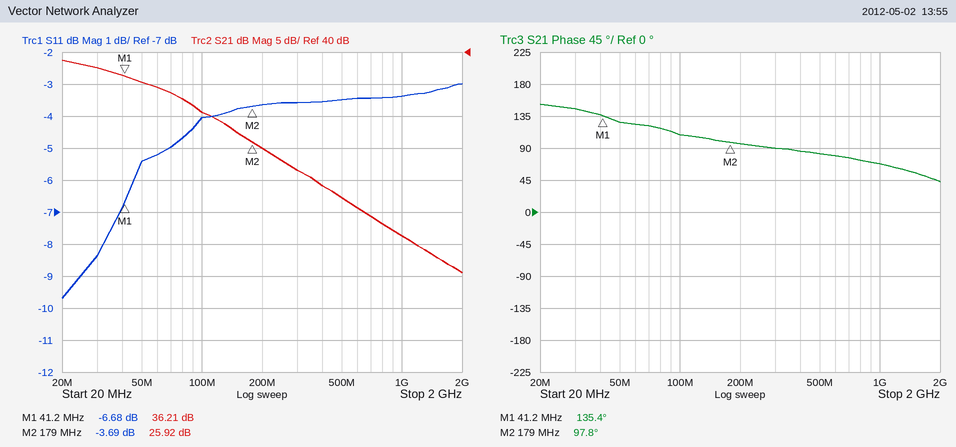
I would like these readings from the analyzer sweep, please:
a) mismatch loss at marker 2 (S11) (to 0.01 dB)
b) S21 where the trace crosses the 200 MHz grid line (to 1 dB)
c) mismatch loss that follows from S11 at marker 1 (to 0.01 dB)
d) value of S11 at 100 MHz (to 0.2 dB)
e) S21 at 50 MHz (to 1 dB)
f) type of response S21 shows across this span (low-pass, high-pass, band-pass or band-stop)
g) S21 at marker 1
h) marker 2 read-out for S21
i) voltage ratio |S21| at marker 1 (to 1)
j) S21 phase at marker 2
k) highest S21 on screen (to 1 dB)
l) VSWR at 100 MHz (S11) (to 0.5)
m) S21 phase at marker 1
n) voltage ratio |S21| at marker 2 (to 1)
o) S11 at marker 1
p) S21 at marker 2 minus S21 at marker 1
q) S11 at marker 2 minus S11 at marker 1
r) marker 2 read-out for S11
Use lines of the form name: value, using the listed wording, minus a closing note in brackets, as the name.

mismatch loss at marker 2 (S11): 2.42 dB
S21 where the trace crosses the 200 MHz grid line: 25 dB
mismatch loss that follows from S11 at marker 1: 1.05 dB
value of S11 at 100 MHz: -4.0 dB
S21 at 50 MHz: 35 dB
type of response S21 shows across this span: low-pass
S21 at marker 1: 36.21 dB
marker 2 read-out for S21: 25.92 dB
voltage ratio |S21| at marker 1: 65
S21 phase at marker 2: 97.8°
highest S21 on screen: 39 dB
VSWR at 100 MHz (S11): 4.5
S21 phase at marker 1: 135.4°
voltage ratio |S21| at marker 2: 20
S11 at marker 1: -6.68 dB
S21 at marker 2 minus S21 at marker 1: -10.29 dB
S11 at marker 2 minus S11 at marker 1: 2.99 dB
marker 2 read-out for S11: -3.69 dB
